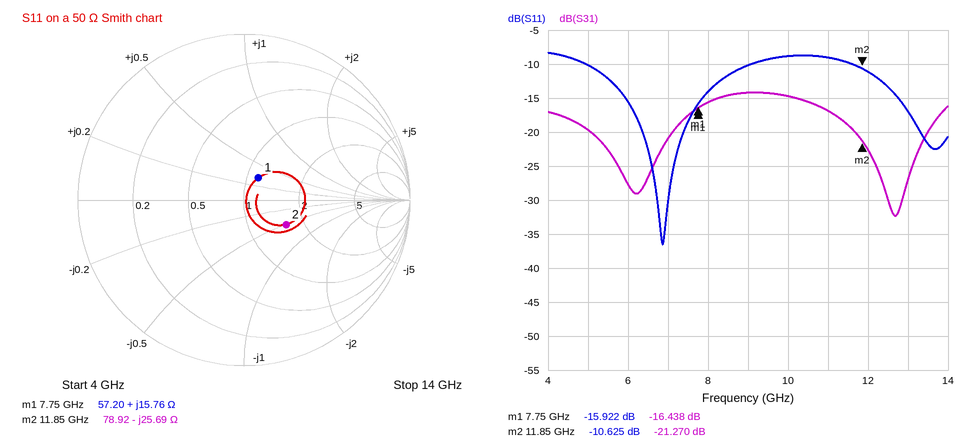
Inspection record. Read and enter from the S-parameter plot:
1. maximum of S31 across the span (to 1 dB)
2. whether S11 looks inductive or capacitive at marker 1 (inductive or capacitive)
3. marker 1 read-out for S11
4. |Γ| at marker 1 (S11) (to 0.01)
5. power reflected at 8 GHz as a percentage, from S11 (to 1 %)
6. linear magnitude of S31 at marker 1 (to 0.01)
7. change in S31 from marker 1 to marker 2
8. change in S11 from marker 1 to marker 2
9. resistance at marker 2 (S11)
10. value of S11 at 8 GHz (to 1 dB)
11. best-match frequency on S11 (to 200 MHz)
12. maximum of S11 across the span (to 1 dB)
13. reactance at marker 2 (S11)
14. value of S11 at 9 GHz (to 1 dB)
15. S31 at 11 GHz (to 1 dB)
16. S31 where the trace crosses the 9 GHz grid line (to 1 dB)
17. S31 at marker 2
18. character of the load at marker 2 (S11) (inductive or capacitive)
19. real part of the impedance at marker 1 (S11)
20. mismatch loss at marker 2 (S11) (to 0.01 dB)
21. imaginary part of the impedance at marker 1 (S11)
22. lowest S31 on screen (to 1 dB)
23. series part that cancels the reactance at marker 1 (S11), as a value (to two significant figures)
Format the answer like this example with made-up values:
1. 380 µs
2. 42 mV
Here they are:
1. -14 dB
2. inductive
3. -15.922 dB
4. 0.16
5. 4 %
6. 0.15
7. -4.832 dB
8. 5.297 dB
9. 78.92 Ω
10. -14 dB
11. 6.8 GHz
12. -8 dB
13. -25.69 Ω
14. -10 dB
15. -17 dB
16. -14 dB
17. -21.270 dB
18. capacitive
19. 57.20 Ω
20. 0.39 dB
21. +15.76 Ω
22. -32 dB
23. 1.3 pF
